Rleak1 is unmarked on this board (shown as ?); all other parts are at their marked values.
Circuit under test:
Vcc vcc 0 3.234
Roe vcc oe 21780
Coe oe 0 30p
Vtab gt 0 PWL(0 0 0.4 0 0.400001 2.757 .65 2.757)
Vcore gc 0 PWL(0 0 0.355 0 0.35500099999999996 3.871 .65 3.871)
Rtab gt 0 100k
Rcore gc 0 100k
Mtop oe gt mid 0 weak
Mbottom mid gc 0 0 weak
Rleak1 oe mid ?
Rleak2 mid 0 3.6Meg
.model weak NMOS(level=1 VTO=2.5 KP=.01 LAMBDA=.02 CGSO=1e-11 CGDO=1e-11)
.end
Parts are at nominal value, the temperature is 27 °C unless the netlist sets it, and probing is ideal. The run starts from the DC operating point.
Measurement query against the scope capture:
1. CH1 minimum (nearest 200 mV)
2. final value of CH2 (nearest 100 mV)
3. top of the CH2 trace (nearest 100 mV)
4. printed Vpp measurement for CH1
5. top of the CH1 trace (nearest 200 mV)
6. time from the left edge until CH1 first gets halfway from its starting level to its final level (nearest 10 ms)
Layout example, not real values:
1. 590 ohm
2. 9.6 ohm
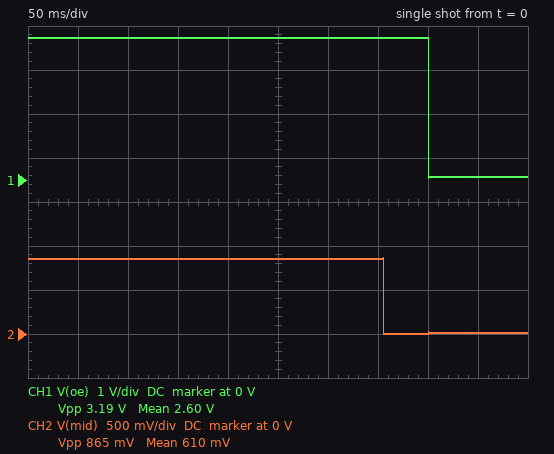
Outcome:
1. 0 V
2. 0 V
3. 900 mV
4. 3.19 V
5. 3.2 V
6. 400 ms
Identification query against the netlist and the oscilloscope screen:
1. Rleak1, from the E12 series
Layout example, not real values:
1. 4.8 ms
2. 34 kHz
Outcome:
1. 10 MΩ
